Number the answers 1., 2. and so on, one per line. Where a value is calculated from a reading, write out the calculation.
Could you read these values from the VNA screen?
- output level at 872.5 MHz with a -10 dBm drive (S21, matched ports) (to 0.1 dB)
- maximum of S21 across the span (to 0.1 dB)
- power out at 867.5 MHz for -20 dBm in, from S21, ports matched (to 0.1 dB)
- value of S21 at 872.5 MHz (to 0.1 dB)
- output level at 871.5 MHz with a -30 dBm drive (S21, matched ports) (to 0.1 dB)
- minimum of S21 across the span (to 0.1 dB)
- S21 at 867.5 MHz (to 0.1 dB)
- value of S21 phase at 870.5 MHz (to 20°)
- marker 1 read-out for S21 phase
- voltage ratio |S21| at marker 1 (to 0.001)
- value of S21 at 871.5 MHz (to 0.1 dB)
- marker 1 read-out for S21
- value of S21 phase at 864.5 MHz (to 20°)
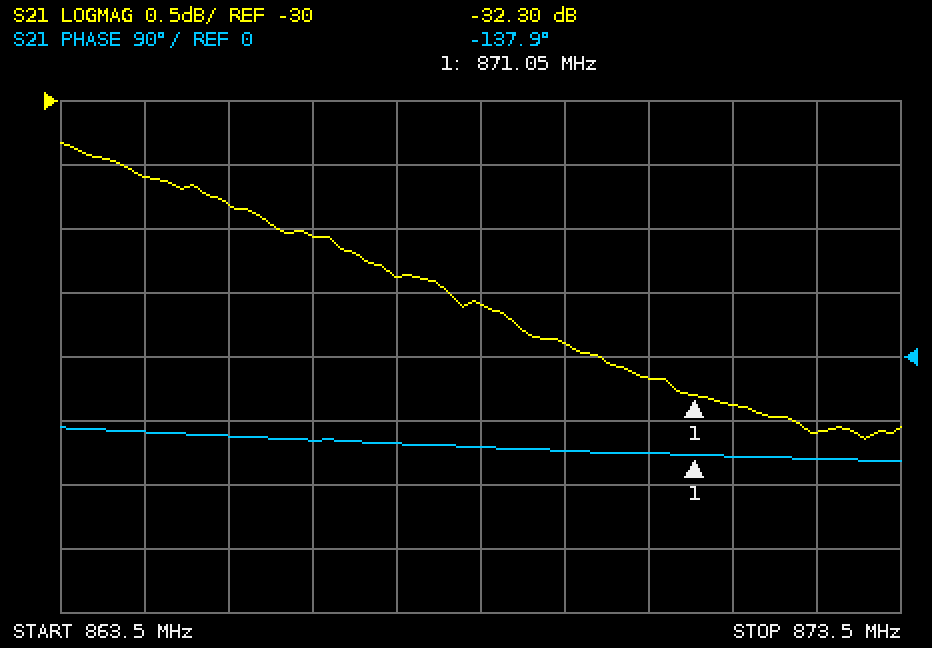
1. -10 dBm + (-32.6 dB) = -42.6 dBm
2. -30.3 dB
3. -20 dBm + (-31.4 dB) = -51.4 dBm
4. -32.6 dB
5. -30 dBm + (-32.4 dB) = -62.4 dBm
6. -32.6 dB
7. -31.4 dB
8. -140°
9. -137.9°
10. 10^(-32.3/20) ≈ 0.024
11. -32.4 dB
12. -32.30 dB
13. -100°
